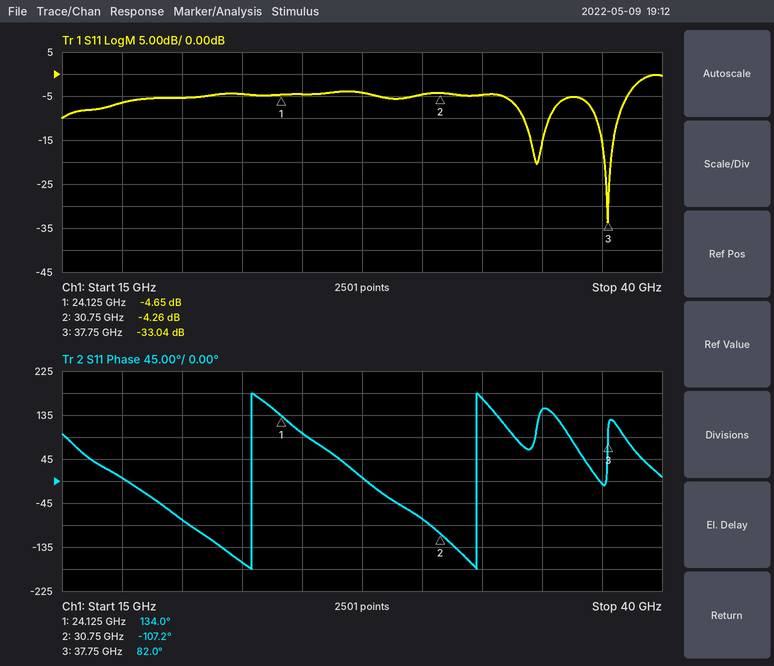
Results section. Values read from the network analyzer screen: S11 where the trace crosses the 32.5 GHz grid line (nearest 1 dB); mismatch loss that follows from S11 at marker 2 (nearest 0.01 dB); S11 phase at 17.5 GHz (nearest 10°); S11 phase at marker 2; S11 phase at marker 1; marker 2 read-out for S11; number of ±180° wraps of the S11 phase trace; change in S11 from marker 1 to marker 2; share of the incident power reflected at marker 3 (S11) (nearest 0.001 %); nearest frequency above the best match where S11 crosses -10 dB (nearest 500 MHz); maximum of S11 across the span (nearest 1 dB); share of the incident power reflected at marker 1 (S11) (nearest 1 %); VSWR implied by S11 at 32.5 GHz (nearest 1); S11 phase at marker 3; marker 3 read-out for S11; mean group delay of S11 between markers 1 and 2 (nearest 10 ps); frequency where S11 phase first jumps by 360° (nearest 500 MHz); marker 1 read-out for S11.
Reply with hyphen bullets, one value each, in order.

- -5 dB
- 2.04 dB
- 10°
- -107.2°
- 134.0°
- -4.26 dB
- 2
- 0.39 dB
- 0.050 %
- 38.0 GHz
- 0 dB
- 34 %
- 4
- 82.0°
- -33.04 dB
- 100 ps
- 23.0 GHz
- -4.65 dB
